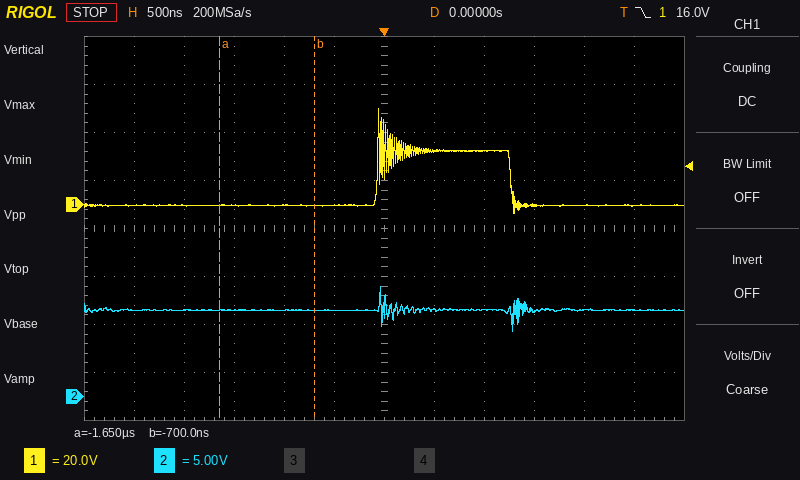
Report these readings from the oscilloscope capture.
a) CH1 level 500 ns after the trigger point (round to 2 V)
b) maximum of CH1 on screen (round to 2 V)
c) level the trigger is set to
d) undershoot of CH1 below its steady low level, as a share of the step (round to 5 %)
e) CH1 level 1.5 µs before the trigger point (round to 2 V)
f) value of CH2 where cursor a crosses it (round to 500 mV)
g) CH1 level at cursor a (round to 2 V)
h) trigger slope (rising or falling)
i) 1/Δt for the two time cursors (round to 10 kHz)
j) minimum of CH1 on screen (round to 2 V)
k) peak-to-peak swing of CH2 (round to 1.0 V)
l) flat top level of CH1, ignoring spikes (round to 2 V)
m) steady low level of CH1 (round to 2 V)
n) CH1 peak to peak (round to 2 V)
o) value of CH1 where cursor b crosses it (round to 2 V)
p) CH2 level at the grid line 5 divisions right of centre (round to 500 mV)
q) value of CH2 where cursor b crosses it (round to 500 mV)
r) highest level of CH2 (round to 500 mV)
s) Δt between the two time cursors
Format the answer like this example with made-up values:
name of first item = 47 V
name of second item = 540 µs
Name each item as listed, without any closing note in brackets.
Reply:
CH1 level 500 ns after the trigger point = 22 V
maximum of CH1 on screen = 40 V
level the trigger is set to = 16.0 V
undershoot of CH1 below its steady low level, as a share of the step = 15 %
CH1 level 1.5 µs before the trigger point = 0 V
value of CH2 where cursor a crosses it = 9.0 V
CH1 level at cursor a = 0 V
trigger slope = falling
1/Δt for the two time cursors = 1.05 MHz
minimum of CH1 on screen = -4 V
peak-to-peak swing of CH2 = 5.0 V
flat top level of CH1, ignoring spikes = 22 V
steady low level of CH1 = 0 V
CH1 peak to peak = 44 V
value of CH1 where cursor b crosses it = 0 V
CH2 level at the grid line 5 divisions right of centre = 9.0 V
value of CH2 where cursor b crosses it = 9.0 V
highest level of CH2 = 11.5 V
Δt between the two time cursors = 950 ns
